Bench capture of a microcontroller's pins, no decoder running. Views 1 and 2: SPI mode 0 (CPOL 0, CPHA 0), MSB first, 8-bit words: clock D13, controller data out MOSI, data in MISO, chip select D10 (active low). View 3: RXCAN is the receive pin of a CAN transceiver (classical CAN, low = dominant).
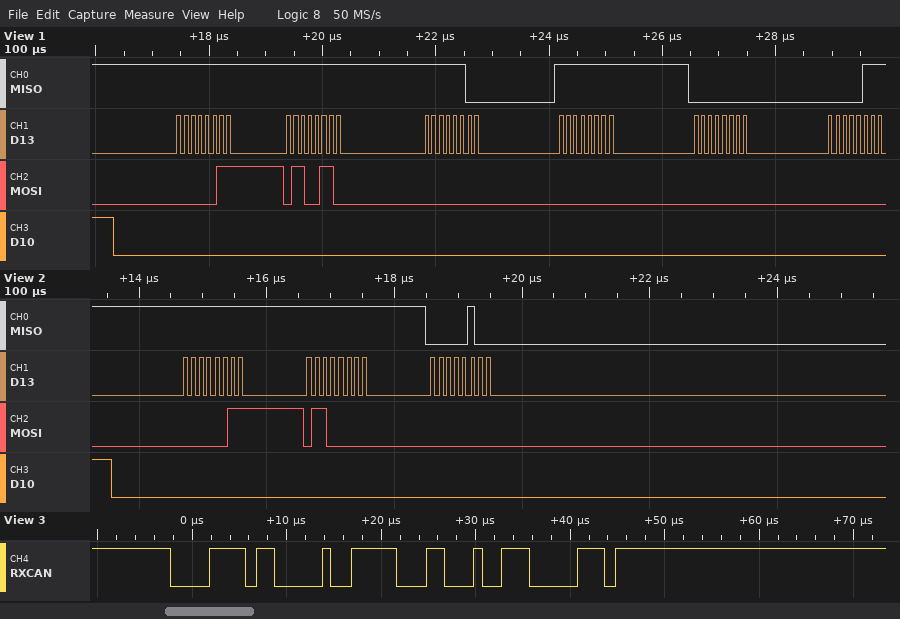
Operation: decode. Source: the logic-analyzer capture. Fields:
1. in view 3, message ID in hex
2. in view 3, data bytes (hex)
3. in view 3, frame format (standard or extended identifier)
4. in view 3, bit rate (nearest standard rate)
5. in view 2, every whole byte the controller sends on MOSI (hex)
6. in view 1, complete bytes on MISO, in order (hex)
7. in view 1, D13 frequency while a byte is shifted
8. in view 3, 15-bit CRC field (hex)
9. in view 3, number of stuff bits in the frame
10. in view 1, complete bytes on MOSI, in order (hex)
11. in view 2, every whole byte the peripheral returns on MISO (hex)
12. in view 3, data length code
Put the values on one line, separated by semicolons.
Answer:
0x0F6; F3; standard; 1000 kbit/s; 0x03 0x60 0x00; 0xFF 0xFF 0xFC 0xFF 0x00 0x07; 8 MHz; 0x09C1; 3; 0x03 0x66 0x00 0x00 0x00 0x00; 0xFF 0xFF 0x04; 1
